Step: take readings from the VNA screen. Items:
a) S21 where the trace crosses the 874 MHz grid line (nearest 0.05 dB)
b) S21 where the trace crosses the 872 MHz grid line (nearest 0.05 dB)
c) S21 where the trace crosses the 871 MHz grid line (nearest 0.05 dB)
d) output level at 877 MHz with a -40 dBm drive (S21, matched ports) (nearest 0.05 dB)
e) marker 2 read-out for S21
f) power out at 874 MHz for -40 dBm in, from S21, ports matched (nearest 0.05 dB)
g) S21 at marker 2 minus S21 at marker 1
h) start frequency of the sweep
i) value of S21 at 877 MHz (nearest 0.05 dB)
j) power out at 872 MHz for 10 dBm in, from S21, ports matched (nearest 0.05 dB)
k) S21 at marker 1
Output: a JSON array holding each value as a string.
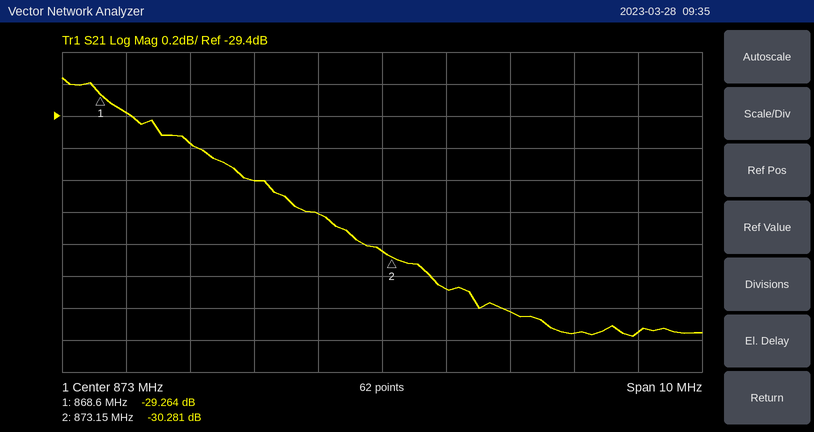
["-30.50 dB", "-30.00 dB", "-29.80 dB", "-70.75 dBm", "-30.281 dB", "-70.50 dBm", "-1.017 dB", "868 MHz", "-30.75 dB", "-20.00 dBm", "-29.264 dB"]
